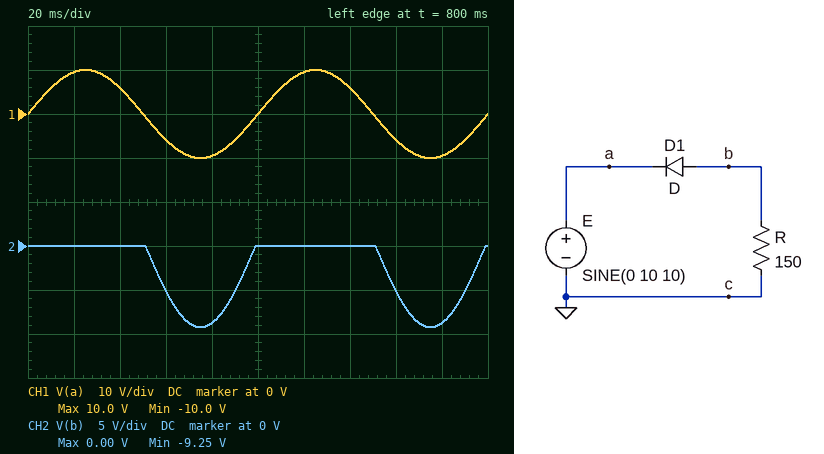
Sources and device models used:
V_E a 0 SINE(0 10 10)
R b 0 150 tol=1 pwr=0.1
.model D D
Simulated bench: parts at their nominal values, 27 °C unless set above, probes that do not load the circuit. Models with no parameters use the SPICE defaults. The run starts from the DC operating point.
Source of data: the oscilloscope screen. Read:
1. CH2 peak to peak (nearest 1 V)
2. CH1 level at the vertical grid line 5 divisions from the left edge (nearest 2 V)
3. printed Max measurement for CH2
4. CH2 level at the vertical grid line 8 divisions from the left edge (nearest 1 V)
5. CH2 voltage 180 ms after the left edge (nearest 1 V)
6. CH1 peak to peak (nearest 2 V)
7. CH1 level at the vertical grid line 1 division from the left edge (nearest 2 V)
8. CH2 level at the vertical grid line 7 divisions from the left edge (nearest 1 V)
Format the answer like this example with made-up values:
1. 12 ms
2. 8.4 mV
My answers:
1. 9 V
2. 0 V
3. 0.00 V
4. -5 V
5. -9 V
6. 20 V
7. 10 V
8. 0 V
